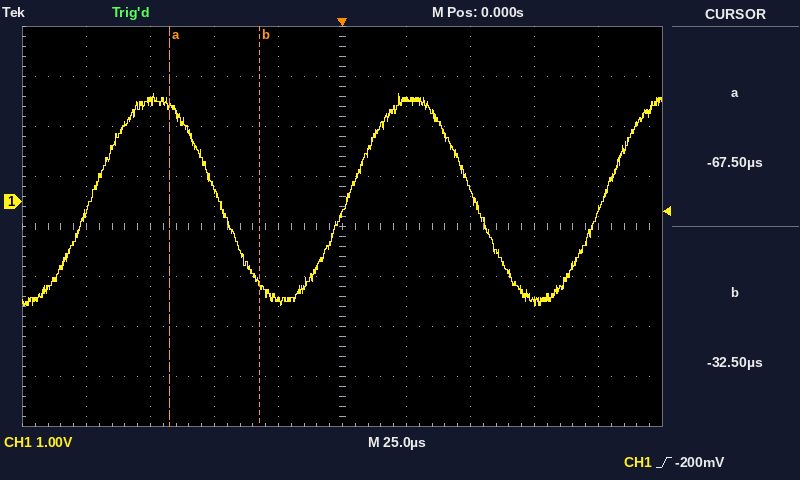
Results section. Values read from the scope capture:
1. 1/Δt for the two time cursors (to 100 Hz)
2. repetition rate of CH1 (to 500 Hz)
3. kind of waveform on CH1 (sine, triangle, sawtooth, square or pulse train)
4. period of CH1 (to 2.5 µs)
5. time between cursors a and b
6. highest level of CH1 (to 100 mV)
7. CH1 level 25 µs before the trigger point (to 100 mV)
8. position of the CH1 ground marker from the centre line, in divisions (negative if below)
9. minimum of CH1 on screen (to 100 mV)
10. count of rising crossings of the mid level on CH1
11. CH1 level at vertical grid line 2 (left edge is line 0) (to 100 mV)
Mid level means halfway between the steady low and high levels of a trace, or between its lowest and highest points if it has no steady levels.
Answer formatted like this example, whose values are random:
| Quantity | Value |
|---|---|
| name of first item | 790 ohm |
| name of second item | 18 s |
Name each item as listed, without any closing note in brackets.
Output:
| Quantity | Value |
|---|---|
| 1/Δt for the two time cursors | 28.6 kHz |
| repetition rate of CH1 | 10.0 kHz |
| kind of waveform on CH1 | sine |
| period of CH1 | 100.0 µs |
| time between cursors a and b | 35.0 µs |
| highest level of CH1 | 2.2 V |
| CH1 level 25 µs before the trigger point | -2.0 V |
| position of the CH1 ground marker from the centre line, in divisions | +0.5 div |
| minimum of CH1 on screen | -2.1 V |
| count of rising crossings of the mid level on CH1 | 3 |
| CH1 level at vertical grid line 2 (left edge is line 0) | 2.0 V |
